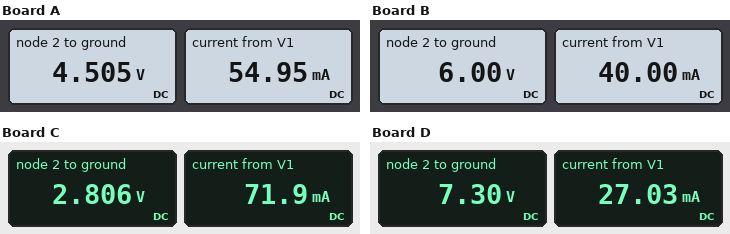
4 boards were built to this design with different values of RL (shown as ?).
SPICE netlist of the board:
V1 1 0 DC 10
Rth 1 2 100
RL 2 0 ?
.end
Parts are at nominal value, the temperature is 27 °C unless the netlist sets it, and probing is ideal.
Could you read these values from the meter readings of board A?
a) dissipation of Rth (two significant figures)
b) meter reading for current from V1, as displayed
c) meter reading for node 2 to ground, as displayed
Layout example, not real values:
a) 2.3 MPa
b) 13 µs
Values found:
a) 300 mW
b) 54.95 mA
c) 4.505 V
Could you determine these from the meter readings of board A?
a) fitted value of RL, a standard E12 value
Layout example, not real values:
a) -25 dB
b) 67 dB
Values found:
a) 82 Ω
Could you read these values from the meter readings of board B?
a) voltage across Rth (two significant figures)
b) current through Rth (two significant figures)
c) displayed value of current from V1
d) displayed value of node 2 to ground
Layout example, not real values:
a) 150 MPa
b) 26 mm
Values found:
a) 4.0 V
b) 40 mA
c) 40.00 mA
d) 6.00 V
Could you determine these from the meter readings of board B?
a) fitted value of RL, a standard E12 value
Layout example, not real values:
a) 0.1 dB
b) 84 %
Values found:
a) 150 Ω
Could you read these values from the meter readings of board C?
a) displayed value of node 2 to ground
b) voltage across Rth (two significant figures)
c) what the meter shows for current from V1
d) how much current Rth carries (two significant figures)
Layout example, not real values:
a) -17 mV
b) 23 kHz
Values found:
a) 2.806 V
b) 7.2 V
c) 71.9 mA
d) 72 mA
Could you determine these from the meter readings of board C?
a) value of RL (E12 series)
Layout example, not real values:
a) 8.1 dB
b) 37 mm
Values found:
a) 39 Ω
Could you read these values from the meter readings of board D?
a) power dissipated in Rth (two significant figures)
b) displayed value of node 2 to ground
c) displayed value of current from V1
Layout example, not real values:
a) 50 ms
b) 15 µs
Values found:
a) 73 mW
b) 7.30 V
c) 27.03 mA
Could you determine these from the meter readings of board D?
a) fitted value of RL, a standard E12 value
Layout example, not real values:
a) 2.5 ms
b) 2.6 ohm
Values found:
a) 270 Ω
